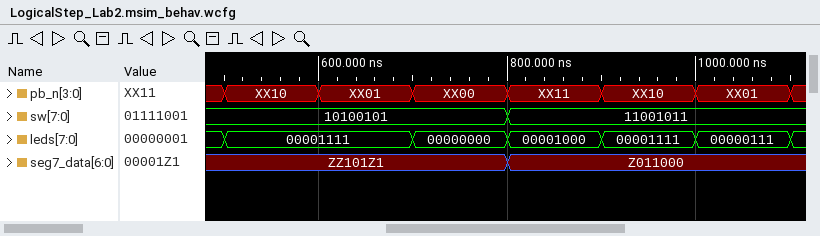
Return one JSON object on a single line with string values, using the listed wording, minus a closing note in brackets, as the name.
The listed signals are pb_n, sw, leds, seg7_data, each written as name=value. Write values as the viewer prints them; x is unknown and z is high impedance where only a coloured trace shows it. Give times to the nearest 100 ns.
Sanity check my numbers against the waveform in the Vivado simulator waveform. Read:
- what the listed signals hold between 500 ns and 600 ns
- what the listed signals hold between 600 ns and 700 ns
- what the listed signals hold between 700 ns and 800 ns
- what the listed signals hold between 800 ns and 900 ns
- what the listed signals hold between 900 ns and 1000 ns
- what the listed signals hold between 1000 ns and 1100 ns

{"what the listed signals hold between 500 ns and 600 ns": "pb_n=XX10, sw=10100101, leds=00001111, seg7_data=ZZ101Z1", "what the listed signals hold between 600 ns and 700 ns": "pb_n=XX01, sw=10100101, leds=00001111, seg7_data=ZZ101Z1", "what the listed signals hold between 700 ns and 800 ns": "pb_n=XX00, sw=10100101, leds=00000000, seg7_data=ZZ101Z1", "what the listed signals hold between 800 ns and 900 ns": "pb_n=XX11, sw=11001011, leds=00001000, seg7_data=Z011000", "what the listed signals hold between 900 ns and 1000 ns": "pb_n=XX10, sw=11001011, leds=00001111, seg7_data=Z011000", "what the listed signals hold between 1000 ns and 1100 ns": "pb_n=XX01, sw=11001011, leds=00000111, seg7_data=Z011000"}
